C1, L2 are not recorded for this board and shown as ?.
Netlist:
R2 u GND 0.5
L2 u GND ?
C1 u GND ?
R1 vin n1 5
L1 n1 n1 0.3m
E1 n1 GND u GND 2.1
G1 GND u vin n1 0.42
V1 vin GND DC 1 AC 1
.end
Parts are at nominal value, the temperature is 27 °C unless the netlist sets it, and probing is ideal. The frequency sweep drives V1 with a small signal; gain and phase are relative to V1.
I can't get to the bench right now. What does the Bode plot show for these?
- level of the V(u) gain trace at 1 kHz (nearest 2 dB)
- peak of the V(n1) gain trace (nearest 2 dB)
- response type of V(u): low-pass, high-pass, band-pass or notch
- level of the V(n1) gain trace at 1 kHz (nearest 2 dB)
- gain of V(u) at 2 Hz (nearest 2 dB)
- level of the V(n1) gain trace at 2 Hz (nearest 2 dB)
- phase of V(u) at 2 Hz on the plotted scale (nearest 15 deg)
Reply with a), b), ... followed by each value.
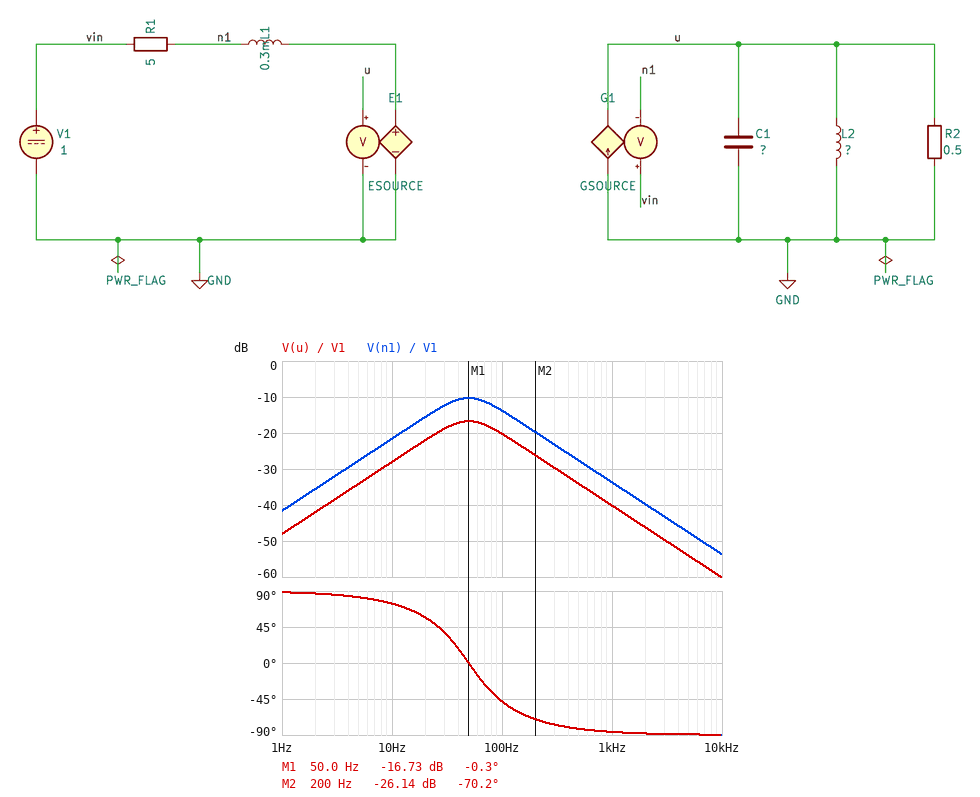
a) -40 dB
b) -10 dB
c) band-pass
d) -34 dB
e) -42 dB
f) -36 dB
g) 90 deg
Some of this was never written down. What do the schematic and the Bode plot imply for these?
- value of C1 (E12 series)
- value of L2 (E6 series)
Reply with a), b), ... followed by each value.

a) 6.8 mF
b) 1.5 mH
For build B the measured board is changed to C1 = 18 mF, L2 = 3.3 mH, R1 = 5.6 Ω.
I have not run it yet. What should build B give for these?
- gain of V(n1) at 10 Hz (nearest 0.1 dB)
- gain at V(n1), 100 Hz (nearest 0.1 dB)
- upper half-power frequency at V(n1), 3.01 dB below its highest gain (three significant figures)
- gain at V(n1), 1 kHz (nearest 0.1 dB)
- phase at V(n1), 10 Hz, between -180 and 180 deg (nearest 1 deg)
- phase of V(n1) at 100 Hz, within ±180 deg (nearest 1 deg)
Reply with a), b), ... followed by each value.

a) -14.5 dB
b) -22.1 dB
c) 37.0 Hz
d) -42.2 dB
e) 52 deg
f) -75 deg
